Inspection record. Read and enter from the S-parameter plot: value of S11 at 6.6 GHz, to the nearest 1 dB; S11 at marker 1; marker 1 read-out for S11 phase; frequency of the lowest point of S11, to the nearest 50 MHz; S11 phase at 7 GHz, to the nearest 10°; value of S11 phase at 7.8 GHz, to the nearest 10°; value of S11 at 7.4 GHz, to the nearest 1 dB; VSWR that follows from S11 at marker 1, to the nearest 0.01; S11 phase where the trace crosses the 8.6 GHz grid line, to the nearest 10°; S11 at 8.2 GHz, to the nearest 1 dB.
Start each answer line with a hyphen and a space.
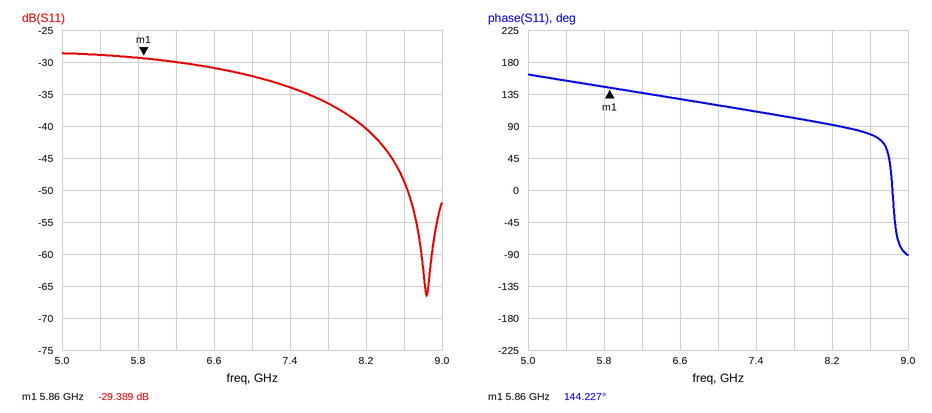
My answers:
- -31 dB
- -29.389 dB
- 144.227°
- 8.85 GHz
- 120°
- 100°
- -34 dB
- 1.07
- 80°
- -40 dB
